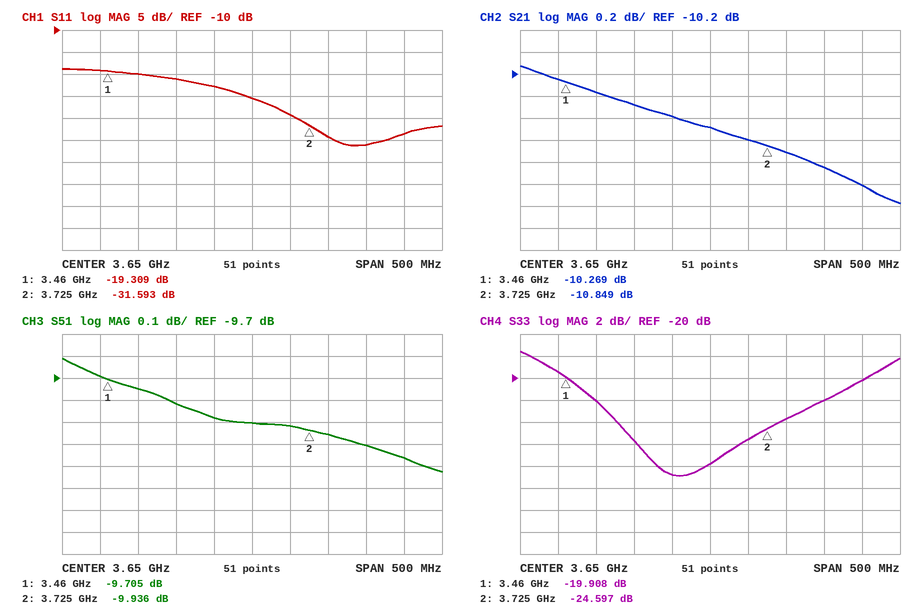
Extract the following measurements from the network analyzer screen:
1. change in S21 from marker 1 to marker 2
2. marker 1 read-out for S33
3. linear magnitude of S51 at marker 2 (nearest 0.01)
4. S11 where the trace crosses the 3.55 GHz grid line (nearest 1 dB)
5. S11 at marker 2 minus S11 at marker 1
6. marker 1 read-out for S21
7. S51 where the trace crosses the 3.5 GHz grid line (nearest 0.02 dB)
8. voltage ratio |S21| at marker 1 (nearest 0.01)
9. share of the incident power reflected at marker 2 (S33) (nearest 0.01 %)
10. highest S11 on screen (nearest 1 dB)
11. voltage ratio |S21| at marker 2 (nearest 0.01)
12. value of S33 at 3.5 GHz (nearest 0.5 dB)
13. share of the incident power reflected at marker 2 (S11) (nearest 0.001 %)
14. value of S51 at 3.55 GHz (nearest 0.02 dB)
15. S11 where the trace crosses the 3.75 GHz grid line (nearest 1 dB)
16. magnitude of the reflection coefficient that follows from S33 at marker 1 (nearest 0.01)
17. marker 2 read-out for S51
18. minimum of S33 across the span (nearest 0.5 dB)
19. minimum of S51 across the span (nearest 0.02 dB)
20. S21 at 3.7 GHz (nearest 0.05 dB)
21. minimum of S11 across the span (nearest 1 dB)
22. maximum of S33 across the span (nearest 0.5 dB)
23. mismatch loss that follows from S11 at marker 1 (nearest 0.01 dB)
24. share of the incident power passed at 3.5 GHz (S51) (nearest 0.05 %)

-0.580 dB
-19.908 dB
0.32
-21 dB
-12.284 dB
-10.269 dB
-9.74 dB
0.31
0.35 %
-19 dB
0.29
-22.0 dB
0.069 %
-9.82 dB
-34 dB
0.10
-9.936 dB
-29.0 dB
-10.12 dB
-10.80 dB
-36 dB
-17.5 dB
0.05 dB
10.60 %
